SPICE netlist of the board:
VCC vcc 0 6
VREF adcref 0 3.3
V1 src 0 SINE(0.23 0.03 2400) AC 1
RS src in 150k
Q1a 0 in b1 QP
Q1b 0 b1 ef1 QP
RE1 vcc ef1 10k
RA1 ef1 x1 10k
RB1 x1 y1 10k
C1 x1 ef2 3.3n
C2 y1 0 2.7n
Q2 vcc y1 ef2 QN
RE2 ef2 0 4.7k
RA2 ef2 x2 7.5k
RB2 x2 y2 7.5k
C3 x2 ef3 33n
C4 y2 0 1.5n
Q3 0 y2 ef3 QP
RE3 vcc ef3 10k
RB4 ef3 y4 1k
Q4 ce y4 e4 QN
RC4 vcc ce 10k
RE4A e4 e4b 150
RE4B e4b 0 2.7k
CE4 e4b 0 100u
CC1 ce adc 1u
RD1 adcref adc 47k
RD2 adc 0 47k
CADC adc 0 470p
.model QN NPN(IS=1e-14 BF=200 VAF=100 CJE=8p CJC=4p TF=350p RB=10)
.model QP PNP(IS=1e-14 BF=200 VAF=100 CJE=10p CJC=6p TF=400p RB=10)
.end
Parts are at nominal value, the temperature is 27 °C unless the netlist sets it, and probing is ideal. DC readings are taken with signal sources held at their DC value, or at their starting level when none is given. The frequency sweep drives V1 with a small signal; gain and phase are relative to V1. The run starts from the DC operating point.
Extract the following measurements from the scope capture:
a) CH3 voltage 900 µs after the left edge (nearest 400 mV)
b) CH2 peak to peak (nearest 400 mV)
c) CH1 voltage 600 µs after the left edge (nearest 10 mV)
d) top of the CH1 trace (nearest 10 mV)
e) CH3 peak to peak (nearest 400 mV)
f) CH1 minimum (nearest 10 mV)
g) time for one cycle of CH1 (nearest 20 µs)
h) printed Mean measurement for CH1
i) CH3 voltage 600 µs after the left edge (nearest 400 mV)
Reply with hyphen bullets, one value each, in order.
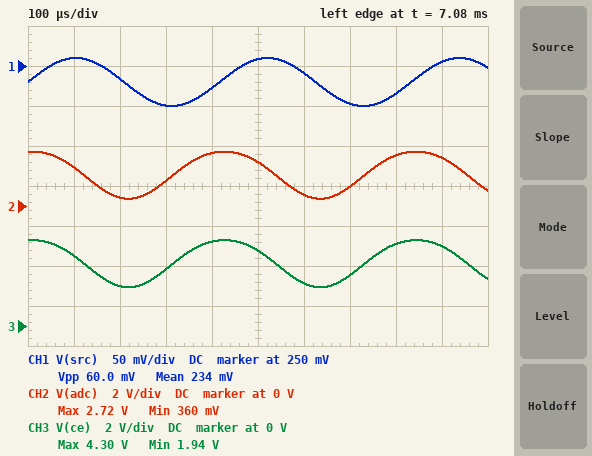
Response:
- 4.0 V
- 2.4 V
- 240 mV
- 260 mV
- 2.4 V
- 200 mV
- 420 µs
- 234 mV
- 2.0 V
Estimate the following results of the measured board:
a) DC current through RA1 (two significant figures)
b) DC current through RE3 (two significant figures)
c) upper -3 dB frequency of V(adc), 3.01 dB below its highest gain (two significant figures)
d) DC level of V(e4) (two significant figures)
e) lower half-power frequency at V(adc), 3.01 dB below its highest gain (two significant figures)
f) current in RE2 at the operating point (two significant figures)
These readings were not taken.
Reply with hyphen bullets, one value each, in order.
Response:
- 740 nA
- 460 µA
- 3.3 kHz
- 790 mV
- 1.3 kHz
- 160 µA
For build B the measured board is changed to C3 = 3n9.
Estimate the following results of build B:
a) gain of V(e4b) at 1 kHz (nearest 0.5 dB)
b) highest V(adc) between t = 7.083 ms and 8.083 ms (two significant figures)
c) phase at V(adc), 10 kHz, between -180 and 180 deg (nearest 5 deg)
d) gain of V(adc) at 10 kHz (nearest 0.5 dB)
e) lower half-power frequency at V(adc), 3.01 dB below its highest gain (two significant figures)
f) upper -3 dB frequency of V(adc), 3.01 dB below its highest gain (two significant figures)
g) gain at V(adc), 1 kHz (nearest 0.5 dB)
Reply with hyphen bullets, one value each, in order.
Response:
- -45.0 dB
- 2.3 V
- -60 deg
- 11.0 dB
- 9.1 Hz
- 3.9 kHz
- 28.0 dB
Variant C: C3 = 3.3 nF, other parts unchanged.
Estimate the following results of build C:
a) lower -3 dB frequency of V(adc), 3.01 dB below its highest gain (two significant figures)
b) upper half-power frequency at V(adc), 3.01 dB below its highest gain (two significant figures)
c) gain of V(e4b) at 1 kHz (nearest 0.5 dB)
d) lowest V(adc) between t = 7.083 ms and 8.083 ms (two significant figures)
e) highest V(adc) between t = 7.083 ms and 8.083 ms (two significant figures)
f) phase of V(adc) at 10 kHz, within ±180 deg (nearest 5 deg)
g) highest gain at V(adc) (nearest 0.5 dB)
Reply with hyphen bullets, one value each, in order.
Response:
- 9.1 Hz
- 3.7 kHz
- -45.0 dB
- 960 mV
- 2.3 V
- -55 deg
- 28.0 dB
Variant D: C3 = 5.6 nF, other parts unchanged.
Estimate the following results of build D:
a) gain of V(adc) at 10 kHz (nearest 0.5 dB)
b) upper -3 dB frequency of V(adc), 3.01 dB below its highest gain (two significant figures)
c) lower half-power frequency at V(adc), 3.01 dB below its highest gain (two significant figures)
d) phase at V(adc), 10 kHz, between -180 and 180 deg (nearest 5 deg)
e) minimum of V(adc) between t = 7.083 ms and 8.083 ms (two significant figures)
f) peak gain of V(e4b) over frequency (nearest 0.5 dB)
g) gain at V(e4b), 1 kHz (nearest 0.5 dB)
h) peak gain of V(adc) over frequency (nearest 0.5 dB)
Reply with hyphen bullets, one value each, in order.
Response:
- 9.5 dB
- 4.3 kHz
- 9.1 Hz
- -80 deg
- 930 mV
- -1.5 dB
- -45.0 dB
- 28.0 dB
